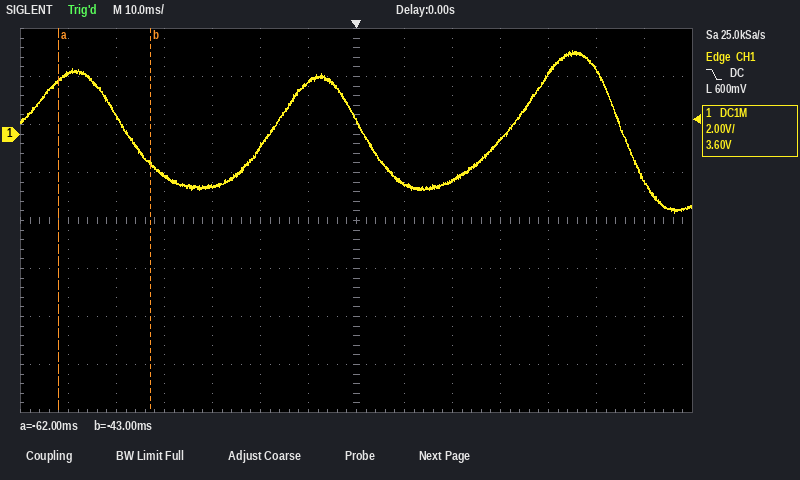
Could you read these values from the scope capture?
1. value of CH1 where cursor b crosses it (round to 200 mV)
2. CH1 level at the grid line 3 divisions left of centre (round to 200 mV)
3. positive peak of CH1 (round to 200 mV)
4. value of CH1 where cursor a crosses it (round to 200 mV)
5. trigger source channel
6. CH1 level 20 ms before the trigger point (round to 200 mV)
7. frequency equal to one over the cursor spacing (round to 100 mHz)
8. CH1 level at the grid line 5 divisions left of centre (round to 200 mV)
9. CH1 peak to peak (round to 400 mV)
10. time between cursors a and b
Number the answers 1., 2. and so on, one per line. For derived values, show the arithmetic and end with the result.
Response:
1. -1.2 V
2. -2.2 V
3. 3.4 V
4. 2.2 V
5. CH1
6. -600 mV
7. 1 / 19 ms ≈ 52.6 Hz
8. 800 mV
9. 6.8 V
10. -43 ms − (-62 ms) = 19 ms
